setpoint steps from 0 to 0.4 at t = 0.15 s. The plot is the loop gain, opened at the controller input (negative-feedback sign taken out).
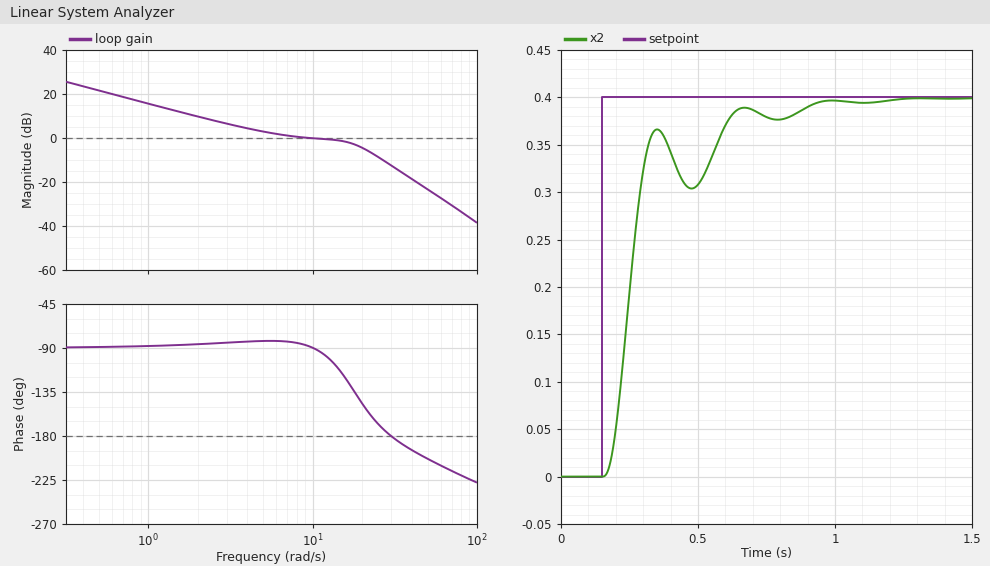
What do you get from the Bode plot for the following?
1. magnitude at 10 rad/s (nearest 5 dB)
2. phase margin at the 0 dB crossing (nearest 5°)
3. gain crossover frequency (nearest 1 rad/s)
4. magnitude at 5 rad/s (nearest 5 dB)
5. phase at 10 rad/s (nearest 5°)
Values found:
0 dB
90°
10 rad/s
5 dB
-90°
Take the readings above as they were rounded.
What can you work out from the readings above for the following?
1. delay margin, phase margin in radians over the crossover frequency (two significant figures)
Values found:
0.16 s
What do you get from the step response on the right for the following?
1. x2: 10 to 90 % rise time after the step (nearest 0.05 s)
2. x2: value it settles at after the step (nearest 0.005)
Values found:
0.15 s
0.400
